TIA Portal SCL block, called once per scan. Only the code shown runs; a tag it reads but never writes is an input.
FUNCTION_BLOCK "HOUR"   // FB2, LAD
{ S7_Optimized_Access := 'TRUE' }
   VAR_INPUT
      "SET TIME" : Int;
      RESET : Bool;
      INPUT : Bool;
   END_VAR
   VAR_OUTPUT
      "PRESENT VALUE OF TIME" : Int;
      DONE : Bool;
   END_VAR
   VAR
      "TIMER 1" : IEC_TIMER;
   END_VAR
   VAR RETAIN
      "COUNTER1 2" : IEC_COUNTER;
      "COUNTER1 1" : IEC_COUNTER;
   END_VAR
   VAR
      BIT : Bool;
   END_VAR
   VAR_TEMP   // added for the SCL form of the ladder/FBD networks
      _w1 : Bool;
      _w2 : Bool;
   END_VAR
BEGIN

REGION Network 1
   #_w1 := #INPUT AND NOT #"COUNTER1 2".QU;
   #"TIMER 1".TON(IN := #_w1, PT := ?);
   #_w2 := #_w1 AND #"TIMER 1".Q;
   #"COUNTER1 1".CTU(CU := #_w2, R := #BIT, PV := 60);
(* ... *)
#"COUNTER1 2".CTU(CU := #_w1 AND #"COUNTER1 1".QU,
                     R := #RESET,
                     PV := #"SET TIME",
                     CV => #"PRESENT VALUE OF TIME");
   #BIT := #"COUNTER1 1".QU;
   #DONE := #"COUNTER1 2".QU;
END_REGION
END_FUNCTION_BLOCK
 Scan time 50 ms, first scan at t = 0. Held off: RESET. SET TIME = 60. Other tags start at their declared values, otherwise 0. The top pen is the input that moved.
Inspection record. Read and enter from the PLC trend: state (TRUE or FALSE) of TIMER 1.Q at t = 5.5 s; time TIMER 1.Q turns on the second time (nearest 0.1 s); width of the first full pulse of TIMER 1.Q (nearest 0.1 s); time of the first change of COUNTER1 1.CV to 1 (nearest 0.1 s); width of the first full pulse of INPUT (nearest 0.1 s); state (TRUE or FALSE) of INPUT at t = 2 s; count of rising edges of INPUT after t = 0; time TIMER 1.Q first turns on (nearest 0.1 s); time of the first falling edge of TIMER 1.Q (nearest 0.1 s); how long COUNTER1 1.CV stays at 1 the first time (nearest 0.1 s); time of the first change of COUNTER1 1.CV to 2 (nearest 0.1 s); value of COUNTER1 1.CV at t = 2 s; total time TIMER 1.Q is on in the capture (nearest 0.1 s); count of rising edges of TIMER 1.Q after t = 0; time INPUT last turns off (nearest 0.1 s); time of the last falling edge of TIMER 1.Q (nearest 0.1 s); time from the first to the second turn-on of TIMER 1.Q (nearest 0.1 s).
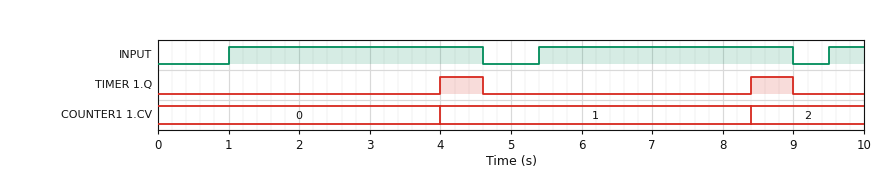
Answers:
FALSE
8.4 s
0.6 s
4.0 s
3.6 s
TRUE
3
4.0 s
4.6 s
4.4 s
8.4 s
0
1.2 s
2
9.0 s
9.0 s
4.4 s
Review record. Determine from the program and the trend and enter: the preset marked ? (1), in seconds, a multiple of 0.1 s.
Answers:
3.0 s
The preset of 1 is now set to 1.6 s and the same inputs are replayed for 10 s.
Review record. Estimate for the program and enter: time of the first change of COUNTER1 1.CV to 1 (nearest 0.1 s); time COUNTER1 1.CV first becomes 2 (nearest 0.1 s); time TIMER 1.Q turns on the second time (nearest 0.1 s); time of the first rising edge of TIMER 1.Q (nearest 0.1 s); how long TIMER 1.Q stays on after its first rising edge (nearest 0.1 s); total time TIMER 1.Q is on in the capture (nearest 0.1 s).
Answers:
2.6 s
7.0 s
7.0 s
2.6 s
2.0 s
4.0 s
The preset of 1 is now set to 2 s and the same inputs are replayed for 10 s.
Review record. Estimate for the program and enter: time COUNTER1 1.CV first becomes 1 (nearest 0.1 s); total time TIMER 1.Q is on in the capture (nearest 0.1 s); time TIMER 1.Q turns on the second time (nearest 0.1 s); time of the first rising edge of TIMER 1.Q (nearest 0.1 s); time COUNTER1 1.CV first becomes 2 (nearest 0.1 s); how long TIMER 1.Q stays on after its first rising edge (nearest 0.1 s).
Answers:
3.0 s
3.2 s
7.4 s
3.0 s
7.4 s
1.6 s
